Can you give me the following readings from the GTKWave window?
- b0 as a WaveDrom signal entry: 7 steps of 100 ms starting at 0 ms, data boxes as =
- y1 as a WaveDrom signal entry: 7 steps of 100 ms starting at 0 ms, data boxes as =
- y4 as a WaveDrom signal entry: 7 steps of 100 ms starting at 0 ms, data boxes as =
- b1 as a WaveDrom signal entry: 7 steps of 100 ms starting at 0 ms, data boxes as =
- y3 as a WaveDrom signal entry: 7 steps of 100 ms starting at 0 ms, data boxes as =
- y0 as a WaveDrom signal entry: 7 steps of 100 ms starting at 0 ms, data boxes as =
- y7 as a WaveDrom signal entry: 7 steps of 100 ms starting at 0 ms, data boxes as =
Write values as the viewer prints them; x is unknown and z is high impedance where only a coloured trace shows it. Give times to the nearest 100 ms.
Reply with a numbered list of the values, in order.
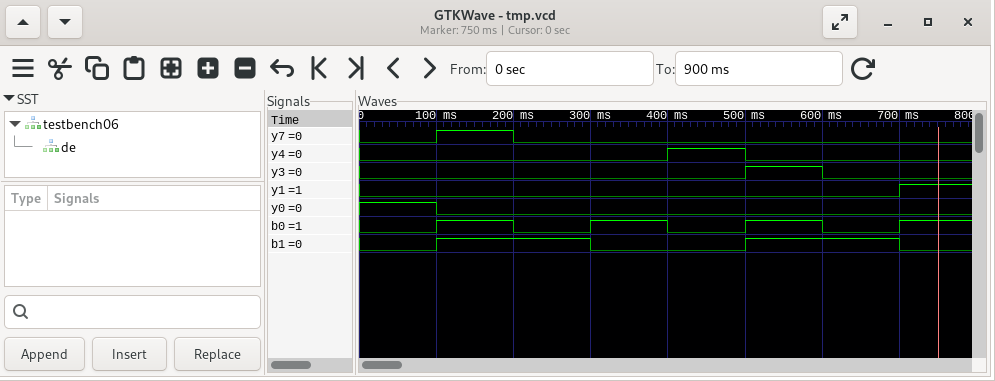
1. {name: 'b0', wave: '0101010'}
2. {name: 'y1', wave: '0......'}
3. {name: 'y4', wave: '0...10.'}
4. {name: 'b1', wave: '01.0.1.'}
5. {name: 'y3', wave: '0....10'}
6. {name: 'y0', wave: '10.....'}
7. {name: 'y7', wave: '010....'}
